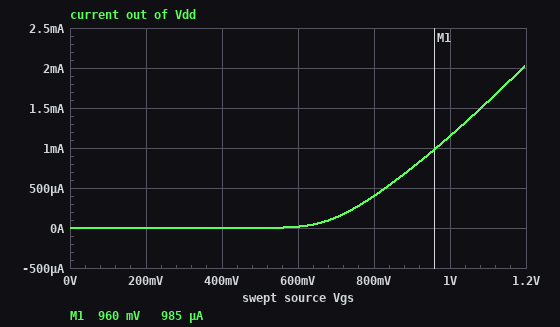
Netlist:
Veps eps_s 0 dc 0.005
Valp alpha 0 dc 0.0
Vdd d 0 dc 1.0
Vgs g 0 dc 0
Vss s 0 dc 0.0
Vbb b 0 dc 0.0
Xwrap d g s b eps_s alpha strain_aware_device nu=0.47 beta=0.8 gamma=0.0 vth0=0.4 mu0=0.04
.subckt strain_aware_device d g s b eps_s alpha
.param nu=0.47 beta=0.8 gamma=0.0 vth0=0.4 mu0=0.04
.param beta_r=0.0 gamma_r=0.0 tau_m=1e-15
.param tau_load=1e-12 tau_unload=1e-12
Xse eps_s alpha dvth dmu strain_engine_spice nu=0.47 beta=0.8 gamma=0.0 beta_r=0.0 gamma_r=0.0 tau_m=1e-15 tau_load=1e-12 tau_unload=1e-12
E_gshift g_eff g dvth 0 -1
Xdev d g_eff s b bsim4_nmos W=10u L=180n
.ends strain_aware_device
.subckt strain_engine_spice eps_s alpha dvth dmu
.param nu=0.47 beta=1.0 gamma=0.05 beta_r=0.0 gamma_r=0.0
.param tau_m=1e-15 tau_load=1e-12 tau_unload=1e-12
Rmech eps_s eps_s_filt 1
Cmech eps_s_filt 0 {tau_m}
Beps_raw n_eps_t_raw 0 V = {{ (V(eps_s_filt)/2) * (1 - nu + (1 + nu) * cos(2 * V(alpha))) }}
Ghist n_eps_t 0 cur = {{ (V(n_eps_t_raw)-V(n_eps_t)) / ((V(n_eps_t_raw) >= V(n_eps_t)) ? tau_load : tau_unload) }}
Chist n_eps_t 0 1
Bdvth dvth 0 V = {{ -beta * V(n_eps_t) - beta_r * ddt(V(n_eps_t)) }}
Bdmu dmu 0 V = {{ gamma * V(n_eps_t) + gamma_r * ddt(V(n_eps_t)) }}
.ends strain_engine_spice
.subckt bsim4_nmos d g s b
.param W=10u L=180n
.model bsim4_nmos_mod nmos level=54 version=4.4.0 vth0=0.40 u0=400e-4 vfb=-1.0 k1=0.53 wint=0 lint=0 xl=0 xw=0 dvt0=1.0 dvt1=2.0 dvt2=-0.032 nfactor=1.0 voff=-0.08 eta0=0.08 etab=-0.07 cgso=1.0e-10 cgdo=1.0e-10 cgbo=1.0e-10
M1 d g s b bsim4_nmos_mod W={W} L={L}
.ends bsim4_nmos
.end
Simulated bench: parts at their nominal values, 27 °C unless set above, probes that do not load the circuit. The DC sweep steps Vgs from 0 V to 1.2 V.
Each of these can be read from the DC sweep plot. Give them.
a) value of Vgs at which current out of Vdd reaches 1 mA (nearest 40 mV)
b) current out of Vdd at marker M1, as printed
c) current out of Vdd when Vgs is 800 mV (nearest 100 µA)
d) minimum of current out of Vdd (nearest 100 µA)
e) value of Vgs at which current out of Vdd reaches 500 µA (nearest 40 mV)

960 mV
985 µA
400 µA
0 A
840 mV
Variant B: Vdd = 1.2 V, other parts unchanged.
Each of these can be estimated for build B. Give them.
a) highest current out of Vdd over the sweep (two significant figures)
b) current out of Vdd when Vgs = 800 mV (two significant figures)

2.1 mA
420 µA
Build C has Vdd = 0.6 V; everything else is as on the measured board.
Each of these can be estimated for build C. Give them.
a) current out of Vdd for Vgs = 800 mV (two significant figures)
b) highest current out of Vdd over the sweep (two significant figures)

350 µA
1.8 mA
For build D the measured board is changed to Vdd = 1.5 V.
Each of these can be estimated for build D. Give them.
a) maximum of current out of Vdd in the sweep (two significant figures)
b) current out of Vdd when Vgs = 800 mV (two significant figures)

2.2 mA
460 µA
